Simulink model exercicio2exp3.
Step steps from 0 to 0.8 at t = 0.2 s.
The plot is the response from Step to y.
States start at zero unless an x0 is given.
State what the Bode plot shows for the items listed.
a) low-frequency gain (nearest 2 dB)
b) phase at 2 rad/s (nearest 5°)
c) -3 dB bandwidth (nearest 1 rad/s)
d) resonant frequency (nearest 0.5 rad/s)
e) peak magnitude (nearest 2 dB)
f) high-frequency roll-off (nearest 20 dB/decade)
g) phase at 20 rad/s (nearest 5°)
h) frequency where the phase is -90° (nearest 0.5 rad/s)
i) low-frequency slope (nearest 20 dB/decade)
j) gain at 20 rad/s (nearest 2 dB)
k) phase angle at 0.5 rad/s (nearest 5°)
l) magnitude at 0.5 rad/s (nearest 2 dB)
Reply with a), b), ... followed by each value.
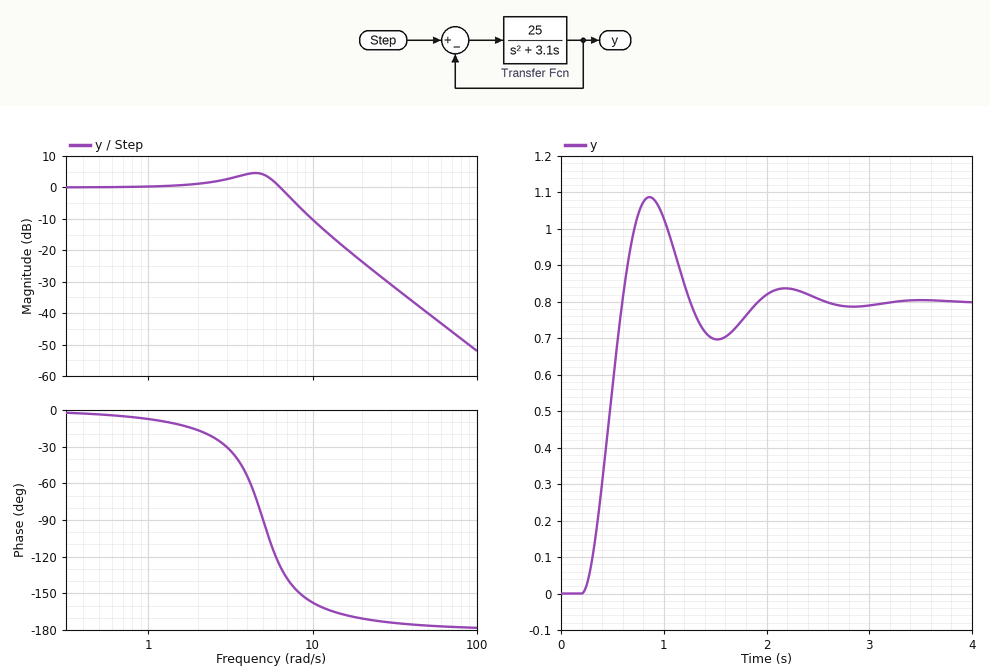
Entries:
a) 0 dB
b) -15°
c) 7 rad/s
d) 4.5 rad/s
e) 4 dB
f) -40 dB/decade
g) -170°
h) 5.0 rad/s
i) 0 dB/decade
j) -24 dB
k) -5°
l) 0 dB
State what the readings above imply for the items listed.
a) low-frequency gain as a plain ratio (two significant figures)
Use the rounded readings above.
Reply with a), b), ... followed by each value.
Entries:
a) 1.0
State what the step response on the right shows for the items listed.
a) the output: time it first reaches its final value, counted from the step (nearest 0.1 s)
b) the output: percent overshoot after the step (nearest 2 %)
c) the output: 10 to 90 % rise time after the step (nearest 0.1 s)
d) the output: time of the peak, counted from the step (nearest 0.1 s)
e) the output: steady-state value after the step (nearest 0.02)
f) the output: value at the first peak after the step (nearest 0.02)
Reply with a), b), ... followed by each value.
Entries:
a) 0.4 s
b) 36 %
c) 0.3 s
d) 0.7 s
e) 0.80
f) 1.08
